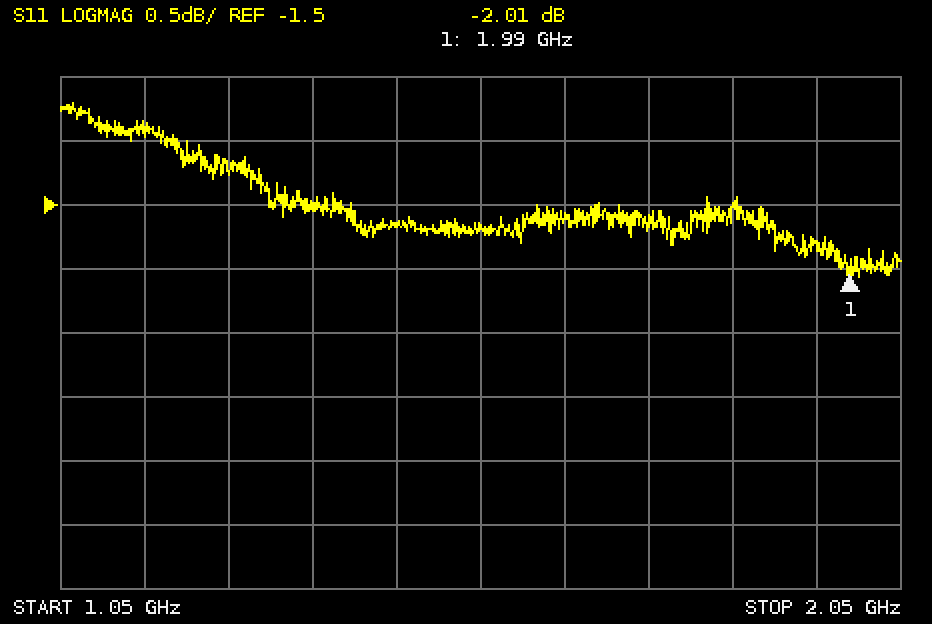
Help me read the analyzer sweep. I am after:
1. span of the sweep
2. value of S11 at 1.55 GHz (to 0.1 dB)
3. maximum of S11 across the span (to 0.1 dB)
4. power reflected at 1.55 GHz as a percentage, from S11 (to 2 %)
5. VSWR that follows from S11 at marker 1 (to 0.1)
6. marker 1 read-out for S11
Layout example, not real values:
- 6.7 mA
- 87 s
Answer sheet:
- 1 GHz
- -1.7 dB
- -0.7 dB
- 68 %
- 8.7
- -2.01 dB
